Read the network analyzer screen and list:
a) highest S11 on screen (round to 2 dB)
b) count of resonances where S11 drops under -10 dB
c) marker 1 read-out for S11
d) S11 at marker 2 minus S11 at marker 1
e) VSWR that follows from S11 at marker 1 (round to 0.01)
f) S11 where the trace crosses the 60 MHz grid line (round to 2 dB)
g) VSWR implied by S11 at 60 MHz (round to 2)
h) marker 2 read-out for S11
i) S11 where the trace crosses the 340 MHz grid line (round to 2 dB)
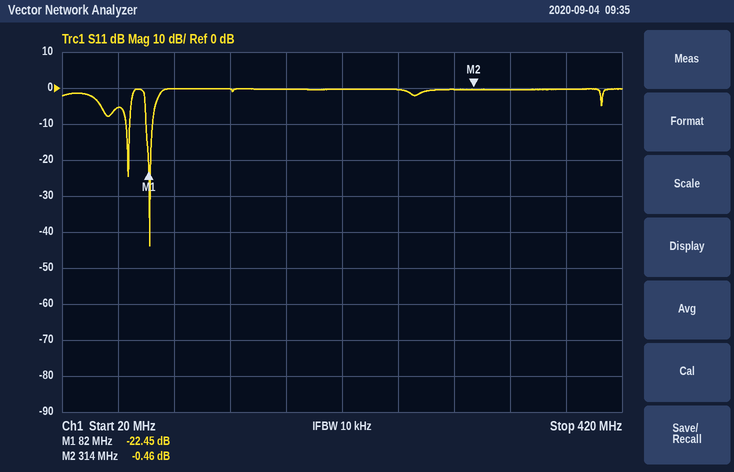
0 dB
2
-22.45 dB
21.99 dB
1.16
-6 dB
4
-0.46 dB
0 dB
